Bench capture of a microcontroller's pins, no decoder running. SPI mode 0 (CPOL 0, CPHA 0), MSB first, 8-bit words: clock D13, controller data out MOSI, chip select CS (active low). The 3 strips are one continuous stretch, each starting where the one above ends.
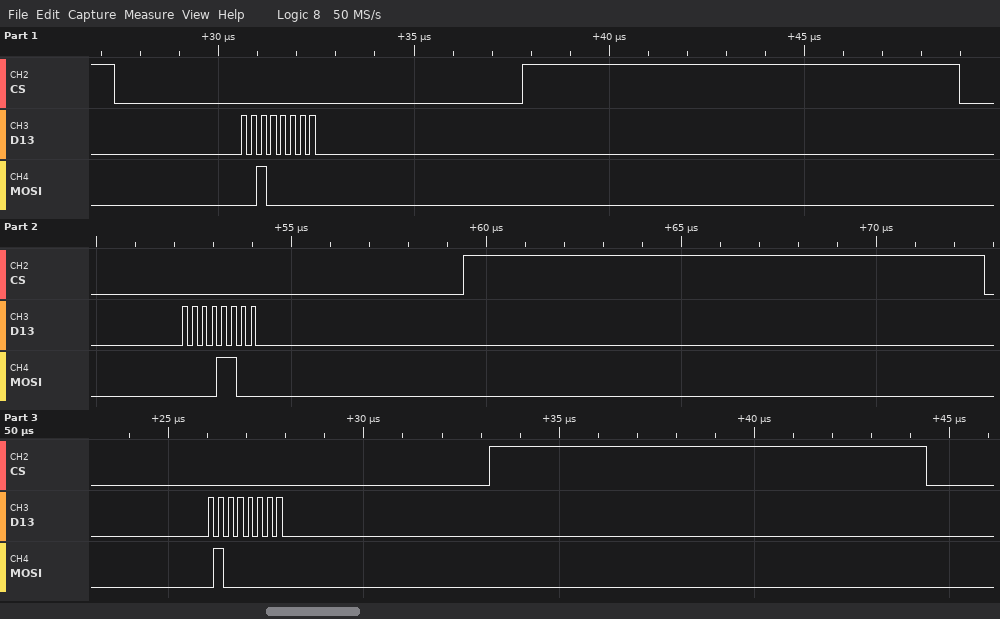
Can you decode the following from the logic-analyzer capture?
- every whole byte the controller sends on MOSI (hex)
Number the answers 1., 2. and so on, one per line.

1. 0x20 0x0C 0x40
